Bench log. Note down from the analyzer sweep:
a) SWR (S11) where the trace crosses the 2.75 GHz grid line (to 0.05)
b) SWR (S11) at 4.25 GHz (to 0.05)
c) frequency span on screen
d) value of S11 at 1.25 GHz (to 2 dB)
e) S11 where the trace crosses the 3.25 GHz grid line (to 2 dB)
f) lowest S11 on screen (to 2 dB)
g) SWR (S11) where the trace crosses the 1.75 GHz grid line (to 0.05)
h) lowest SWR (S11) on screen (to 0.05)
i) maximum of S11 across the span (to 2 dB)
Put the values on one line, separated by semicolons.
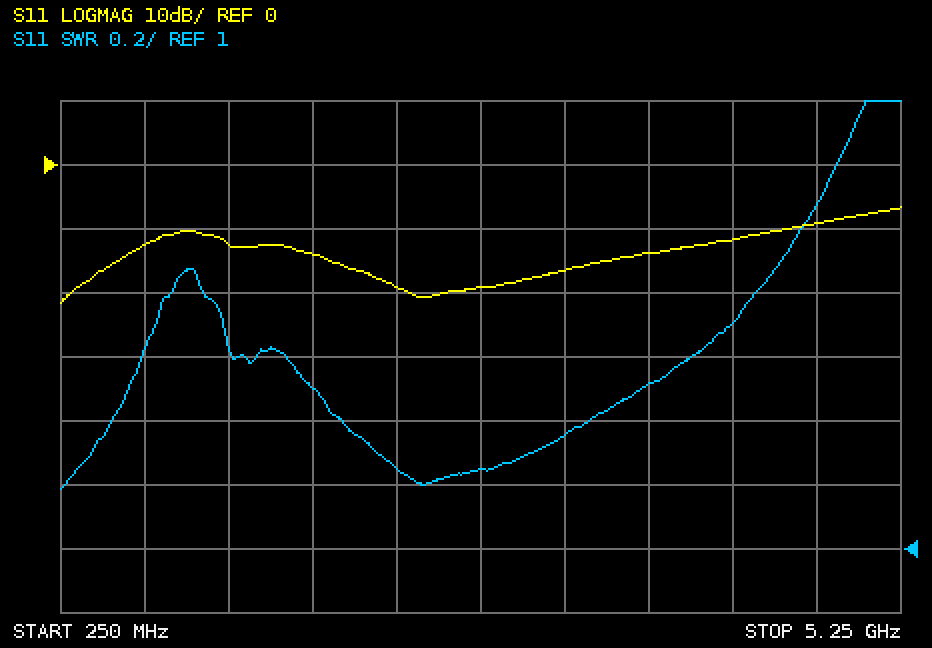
1.25; 1.70; 5 GHz; -12 dB; -16 dB; -22 dB; 1.50; 1.20; -6 dB
